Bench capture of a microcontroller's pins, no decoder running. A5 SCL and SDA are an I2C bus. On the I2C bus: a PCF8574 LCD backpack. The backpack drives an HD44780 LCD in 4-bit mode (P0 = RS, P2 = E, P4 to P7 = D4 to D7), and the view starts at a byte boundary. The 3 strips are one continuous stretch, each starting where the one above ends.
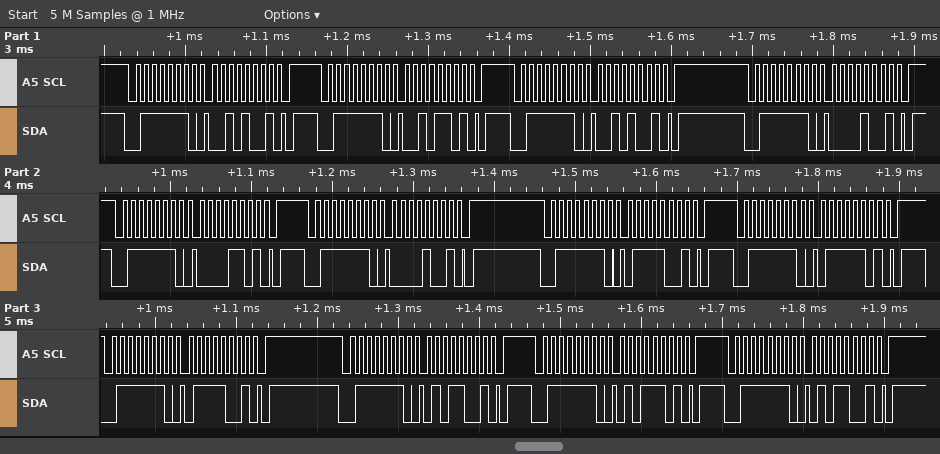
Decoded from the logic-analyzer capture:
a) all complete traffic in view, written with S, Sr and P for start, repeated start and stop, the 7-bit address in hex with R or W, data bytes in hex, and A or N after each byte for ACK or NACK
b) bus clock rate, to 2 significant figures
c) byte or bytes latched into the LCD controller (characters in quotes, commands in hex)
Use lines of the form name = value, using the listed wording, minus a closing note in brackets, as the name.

all complete traffic in view, written with S, Sr and P for start, repeated start and stop, the 7-bit address in hex with R or W, data bytes in hex, and A or N after each byte for ACK or NACK = S 3FW A 29 A P S 3FW A 2D A P S 3FW A 29 A P S 3FW A 09 A P S 3FW A 0D A P S 3FW A 09 A P S 3FW A 79 A P S 3FW A 7D A P S 3FW A 79 A P S 3FW A 59 A P S 3FW A 5D A P S 3FW A 59 A P
bus clock rate, to 2 significant figures = 100 kHz
byte or bytes latched into the LCD controller = ' ' 'u'
